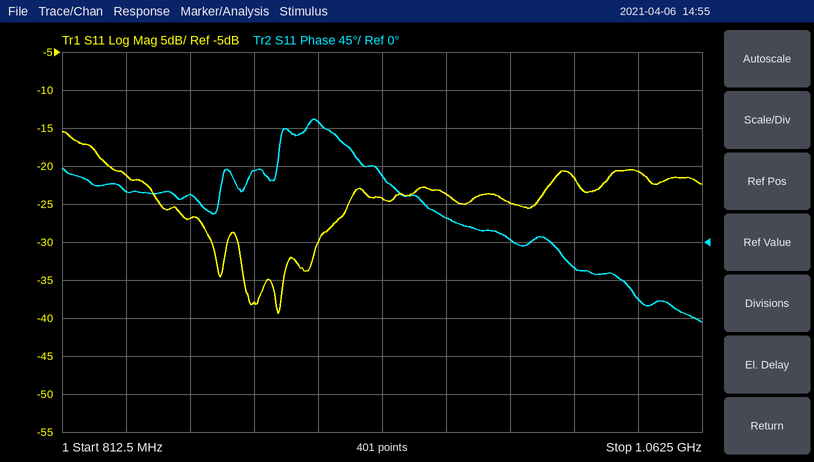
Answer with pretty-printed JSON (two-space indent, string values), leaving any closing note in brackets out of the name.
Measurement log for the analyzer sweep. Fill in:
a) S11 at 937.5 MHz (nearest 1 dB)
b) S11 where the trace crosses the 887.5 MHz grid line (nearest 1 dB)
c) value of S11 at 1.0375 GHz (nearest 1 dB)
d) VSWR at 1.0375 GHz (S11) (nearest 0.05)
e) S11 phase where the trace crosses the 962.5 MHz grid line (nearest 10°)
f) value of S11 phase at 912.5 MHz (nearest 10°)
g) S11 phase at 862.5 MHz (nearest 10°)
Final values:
{
  "S11 at 937.5 MHz": "-24 dB",
  "S11 where the trace crosses the 887.5 MHz grid line": "-38 dB",
  "value of S11 at 1.0375 GHz": "-21 dB",
  "VSWR at 1.0375 GHz (S11)": "1.20",
  "S11 phase where the trace crosses the 962.5 MHz grid line": "30°",
  "value of S11 phase at 912.5 MHz": "140°",
  "S11 phase at 862.5 MHz": "60°"
}
